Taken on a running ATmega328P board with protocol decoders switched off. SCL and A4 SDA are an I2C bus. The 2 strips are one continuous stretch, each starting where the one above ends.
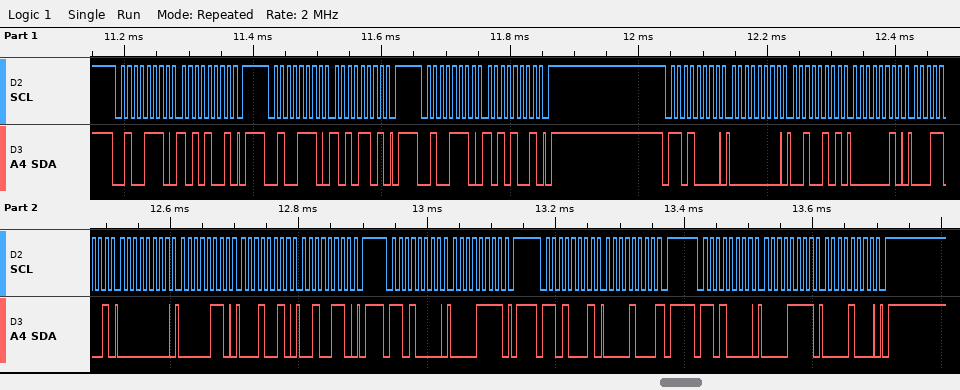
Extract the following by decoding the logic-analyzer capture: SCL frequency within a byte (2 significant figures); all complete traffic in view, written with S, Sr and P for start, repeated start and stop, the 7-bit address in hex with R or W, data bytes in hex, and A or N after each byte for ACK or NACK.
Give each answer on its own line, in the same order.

100 kHz
S 27W A A9 A P S 27W A AD A P S 27W A A9 A P S 68W A 00 A 25 A 02 A 19 A 00 A 06 A 12 A 26 A P S 68W A 0F A P S 68R A 08 N P S 68W A 0F A 08 A P
